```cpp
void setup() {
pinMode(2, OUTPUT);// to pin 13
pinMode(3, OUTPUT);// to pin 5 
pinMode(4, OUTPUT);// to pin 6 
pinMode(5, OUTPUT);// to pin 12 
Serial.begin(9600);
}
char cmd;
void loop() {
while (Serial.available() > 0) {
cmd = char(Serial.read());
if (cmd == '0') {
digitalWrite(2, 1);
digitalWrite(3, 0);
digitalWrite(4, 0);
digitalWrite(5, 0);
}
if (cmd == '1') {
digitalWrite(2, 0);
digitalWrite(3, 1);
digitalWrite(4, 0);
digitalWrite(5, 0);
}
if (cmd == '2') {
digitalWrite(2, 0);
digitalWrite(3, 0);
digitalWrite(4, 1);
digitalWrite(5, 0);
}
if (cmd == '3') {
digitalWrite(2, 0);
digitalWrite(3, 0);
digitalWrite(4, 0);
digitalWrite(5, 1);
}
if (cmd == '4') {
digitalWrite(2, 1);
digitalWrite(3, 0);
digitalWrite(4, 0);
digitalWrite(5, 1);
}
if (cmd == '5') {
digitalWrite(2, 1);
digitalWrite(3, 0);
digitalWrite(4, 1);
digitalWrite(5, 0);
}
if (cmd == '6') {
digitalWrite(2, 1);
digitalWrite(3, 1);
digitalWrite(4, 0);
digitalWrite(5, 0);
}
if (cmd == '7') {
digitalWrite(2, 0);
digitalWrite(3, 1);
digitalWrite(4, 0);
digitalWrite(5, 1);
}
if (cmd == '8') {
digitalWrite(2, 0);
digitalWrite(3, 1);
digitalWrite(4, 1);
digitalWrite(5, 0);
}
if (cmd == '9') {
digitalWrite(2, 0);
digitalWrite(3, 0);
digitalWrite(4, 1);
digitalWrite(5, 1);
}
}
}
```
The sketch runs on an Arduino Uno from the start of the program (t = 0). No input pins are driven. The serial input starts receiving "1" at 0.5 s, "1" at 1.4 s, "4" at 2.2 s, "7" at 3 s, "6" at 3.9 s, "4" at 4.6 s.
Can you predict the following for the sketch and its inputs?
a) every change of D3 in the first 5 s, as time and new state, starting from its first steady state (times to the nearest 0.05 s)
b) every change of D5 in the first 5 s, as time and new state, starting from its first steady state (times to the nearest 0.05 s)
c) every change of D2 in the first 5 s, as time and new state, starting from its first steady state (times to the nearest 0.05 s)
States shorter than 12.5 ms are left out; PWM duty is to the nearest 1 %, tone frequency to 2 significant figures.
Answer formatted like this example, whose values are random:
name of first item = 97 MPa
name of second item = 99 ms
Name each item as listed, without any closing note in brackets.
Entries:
every change of D3 in the first 5 s, as time and new state, starting from its first steady state = 0 s low; 0.5 s high; 2.2 s low; 3 s high; 4.6 s low
every change of D5 in the first 5 s, as time and new state, starting from its first steady state = 0 s low; 2.2 s high; 3.9 s low; 4.6 s high
every change of D2 in the first 5 s, as time and new state, starting from its first steady state = 0 s low; 2.2 s high; 3 s low; 3.9 s high
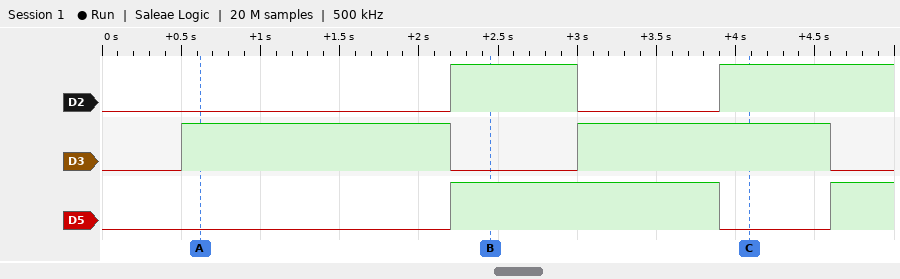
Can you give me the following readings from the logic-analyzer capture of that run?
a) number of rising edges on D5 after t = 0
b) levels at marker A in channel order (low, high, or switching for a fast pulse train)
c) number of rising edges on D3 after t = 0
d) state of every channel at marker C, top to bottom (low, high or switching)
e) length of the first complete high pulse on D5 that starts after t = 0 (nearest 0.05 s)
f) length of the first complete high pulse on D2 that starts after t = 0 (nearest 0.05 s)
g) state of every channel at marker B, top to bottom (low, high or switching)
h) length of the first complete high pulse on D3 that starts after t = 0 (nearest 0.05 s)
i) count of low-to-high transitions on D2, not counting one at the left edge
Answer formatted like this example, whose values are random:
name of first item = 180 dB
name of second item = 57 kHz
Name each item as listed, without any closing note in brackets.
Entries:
number of rising edges on D5 after t = 0 = 2
levels at marker A in channel order = D2 low, D3 high, D5 low
number of rising edges on D3 after t = 0 = 2
state of every channel at marker C, top to bottom = D2 high, D3 high, D5 low
length of the first complete high pulse on D5 that starts after t = 0 = 1.70 s
length of the first complete high pulse on D2 that starts after t = 0 = 0.80 s
state of every channel at marker B, top to bottom = D2 high, D3 low, D5 high
length of the first complete high pulse on D3 that starts after t = 0 = 1.70 s
count of low-to-high transitions on D2, not counting one at the left edge = 2
